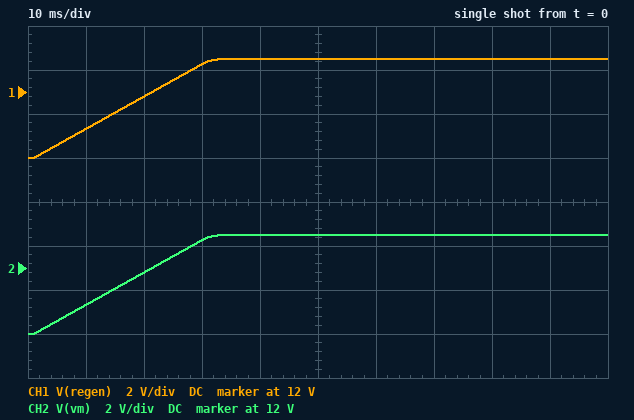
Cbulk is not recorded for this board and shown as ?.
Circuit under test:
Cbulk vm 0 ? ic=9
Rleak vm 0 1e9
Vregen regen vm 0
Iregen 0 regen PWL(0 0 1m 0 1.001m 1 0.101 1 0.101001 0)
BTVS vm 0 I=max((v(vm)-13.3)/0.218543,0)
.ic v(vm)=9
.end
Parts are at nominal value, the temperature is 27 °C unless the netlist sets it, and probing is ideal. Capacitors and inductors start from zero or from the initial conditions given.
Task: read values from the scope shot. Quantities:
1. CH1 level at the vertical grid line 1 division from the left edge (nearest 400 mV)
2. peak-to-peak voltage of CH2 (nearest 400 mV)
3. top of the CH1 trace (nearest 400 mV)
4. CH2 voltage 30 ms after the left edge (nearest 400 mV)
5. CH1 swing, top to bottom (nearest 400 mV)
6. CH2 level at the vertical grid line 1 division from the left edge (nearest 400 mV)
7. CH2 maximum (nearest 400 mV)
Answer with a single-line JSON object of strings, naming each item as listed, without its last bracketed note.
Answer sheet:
{"CH1 level at the vertical grid line 1 division from the left edge": "10.4 V", "peak-to-peak voltage of CH2": "4.4 V", "top of the CH1 trace": "13.6 V", "CH2 voltage 30 ms after the left edge": "13.2 V", "CH1 swing, top to bottom": "4.4 V", "CH2 level at the vertical grid line 1 division from the left edge": "10.4 V", "CH2 maximum": "13.6 V"}
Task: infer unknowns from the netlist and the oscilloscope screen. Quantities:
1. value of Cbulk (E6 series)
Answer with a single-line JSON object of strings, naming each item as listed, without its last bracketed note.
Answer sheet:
{"value of Cbulk": "6.8 mF"}
